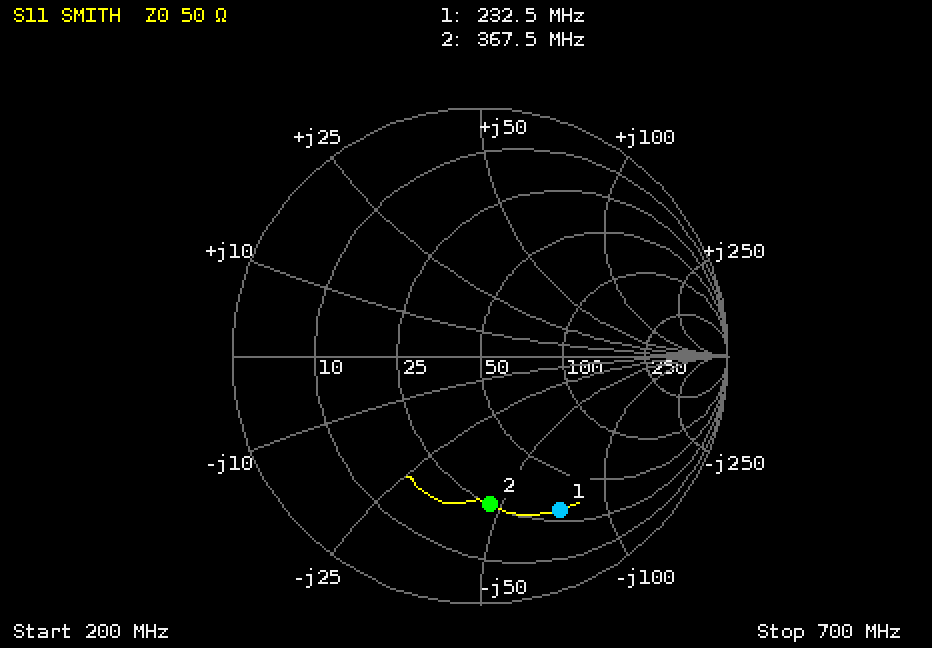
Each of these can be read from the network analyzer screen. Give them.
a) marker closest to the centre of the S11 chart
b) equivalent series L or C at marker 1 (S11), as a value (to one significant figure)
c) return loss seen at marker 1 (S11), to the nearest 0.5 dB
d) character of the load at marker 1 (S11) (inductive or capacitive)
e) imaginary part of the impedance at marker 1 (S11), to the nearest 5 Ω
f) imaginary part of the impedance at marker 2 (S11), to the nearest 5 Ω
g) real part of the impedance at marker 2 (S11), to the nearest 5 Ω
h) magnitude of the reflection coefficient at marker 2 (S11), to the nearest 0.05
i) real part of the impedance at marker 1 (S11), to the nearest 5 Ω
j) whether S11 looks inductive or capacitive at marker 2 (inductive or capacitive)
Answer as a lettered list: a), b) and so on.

a) marker 2
b) 9 pF
c) 3.0 dB
d) capacitive
e) -75 Ω
f) -45 Ω
g) 25 Ω
h) 0.60
i) 30 Ω
j) capacitive
